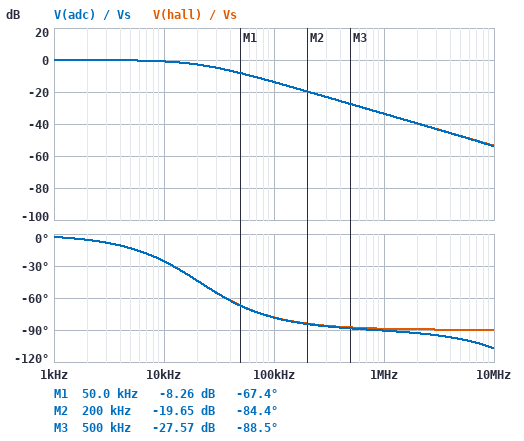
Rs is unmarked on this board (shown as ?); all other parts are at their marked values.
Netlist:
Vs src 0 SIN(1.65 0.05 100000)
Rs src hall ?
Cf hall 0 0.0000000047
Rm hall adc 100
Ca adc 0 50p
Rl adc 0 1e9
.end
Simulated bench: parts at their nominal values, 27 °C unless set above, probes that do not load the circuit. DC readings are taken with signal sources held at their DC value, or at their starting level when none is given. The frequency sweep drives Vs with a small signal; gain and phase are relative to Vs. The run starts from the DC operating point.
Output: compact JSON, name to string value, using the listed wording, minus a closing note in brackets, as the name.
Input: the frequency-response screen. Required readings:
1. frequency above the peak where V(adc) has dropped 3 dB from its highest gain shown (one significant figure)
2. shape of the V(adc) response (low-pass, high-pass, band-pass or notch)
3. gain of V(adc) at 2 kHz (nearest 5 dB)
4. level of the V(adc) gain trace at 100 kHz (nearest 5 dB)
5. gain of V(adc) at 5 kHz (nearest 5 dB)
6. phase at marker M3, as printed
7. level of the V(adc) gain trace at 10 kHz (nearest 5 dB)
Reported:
{"frequency above the peak where V(adc) has dropped 3 dB from its highest gain shown": "20 kHz", "shape of the V(adc) response": "low-pass", "gain of V(adc) at 2 kHz": "0 dB", "level of the V(adc) gain trace at 100 kHz": "-15 dB", "gain of V(adc) at 5 kHz": "0 dB", "phase at marker M3, as printed": "-88.5 deg", "level of the V(adc) gain trace at 10 kHz": "0 dB"}
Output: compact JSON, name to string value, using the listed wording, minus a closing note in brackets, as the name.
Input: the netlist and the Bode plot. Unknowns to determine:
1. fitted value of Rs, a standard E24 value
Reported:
{"fitted value of Rs, a standard E24 value": "1.6 kΩ"}
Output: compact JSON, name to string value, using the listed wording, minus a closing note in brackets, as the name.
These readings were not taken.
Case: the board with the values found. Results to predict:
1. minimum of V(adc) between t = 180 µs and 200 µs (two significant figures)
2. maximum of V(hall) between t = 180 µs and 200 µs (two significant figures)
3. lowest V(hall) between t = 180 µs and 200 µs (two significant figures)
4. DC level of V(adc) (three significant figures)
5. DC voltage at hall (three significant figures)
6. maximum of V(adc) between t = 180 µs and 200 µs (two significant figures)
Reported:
{"minimum of V(adc) between t = 180 µs and 200 µs": "1.6 V", "maximum of V(hall) between t = 180 µs and 200 µs": "1.7 V", "lowest V(hall) between t = 180 µs and 200 µs": "1.6 V", "DC level of V(adc)": "1.65 V", "DC voltage at hall": "1.65 V", "maximum of V(adc) between t = 180 µs and 200 µs": "1.7 V"}
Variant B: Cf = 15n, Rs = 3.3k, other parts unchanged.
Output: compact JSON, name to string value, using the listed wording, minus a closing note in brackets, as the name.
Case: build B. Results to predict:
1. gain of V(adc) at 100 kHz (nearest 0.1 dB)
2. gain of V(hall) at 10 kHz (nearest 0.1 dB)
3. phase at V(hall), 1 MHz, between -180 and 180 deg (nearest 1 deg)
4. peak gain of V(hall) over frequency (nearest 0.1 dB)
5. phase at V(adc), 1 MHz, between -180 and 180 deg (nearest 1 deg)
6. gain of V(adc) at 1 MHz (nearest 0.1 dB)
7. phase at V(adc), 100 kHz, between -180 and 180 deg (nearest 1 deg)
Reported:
{"gain of V(adc) at 100 kHz": "-29.9 dB", "gain of V(hall) at 10 kHz": "-10.3 dB", "phase at V(hall), 1 MHz, between -180 and 180 deg": "-90 deg", "peak gain of V(hall) over frequency": "0 dB", "phase at V(adc), 1 MHz, between -180 and 180 deg": "-92 deg", "gain of V(adc) at 1 MHz": "-49.9 dB", "phase at V(adc), 100 kHz, between -180 and 180 deg": "-88 deg"}
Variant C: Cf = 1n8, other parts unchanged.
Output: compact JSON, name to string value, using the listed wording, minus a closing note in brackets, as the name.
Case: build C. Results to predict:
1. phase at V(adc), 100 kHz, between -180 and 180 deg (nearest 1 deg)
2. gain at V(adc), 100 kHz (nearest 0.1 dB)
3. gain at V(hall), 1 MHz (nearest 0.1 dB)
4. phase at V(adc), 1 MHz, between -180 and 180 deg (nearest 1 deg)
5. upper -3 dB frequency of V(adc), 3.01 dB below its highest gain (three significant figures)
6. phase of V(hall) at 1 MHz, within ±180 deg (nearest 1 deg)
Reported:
{"phase at V(adc), 100 kHz, between -180 and 180 deg": "-62 deg", "gain at V(adc), 100 kHz": "-6.5 dB", "gain at V(hall), 1 MHz": "-25.4 dB", "phase at V(adc), 1 MHz, between -180 and 180 deg": "-89 deg", "upper -3 dB frequency of V(adc), 3.01 dB below its highest gain": "53.8 kHz", "phase of V(hall) at 1 MHz, within ±180 deg": "-87 deg"}
